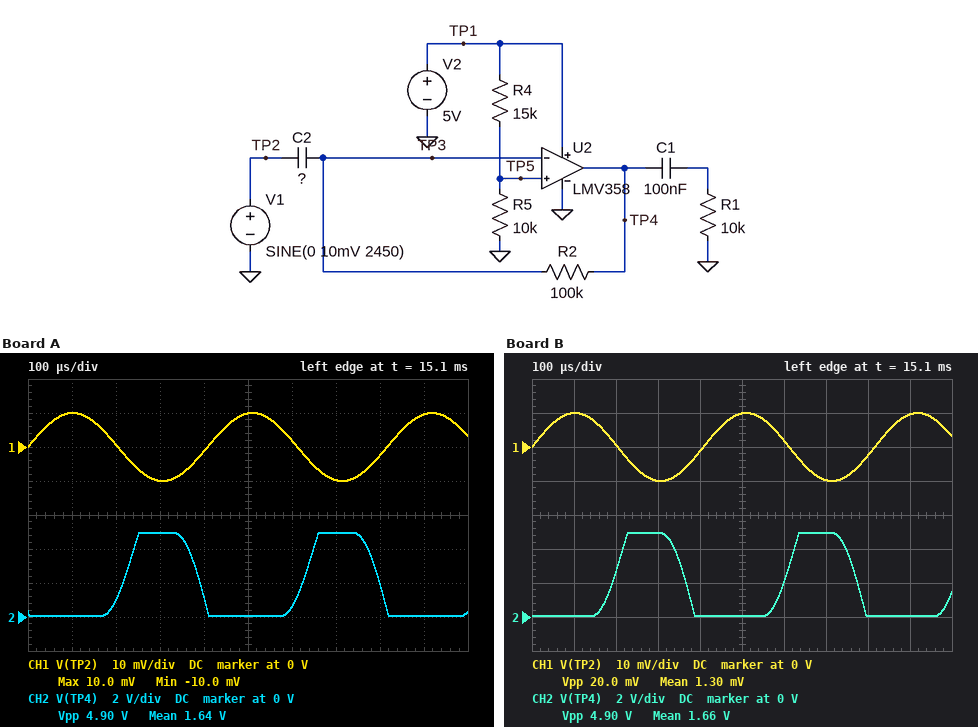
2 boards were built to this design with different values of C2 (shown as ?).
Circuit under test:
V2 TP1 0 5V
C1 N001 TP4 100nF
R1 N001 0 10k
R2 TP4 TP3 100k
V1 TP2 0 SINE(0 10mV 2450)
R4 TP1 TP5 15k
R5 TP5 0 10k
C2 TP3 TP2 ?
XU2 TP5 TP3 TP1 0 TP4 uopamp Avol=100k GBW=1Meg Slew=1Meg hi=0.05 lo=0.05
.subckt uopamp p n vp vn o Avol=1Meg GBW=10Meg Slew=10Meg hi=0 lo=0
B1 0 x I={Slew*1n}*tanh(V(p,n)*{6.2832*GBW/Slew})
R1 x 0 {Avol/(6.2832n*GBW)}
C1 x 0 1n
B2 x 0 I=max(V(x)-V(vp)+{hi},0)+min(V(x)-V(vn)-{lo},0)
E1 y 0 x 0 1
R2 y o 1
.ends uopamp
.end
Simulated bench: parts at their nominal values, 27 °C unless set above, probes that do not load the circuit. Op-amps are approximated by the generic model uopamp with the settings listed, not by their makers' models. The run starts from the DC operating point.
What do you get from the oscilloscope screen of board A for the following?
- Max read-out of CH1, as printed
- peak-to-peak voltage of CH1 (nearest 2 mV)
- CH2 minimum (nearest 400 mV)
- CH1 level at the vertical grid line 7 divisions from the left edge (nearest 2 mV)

10.0 mV
20 mV
0 V
-10 mV
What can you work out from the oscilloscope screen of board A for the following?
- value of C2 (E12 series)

150 nF
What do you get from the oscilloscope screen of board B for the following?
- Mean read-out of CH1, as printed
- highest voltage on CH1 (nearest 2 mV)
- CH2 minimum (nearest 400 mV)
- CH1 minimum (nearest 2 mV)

1.30 mV
10 mV
0 V
-10 mV
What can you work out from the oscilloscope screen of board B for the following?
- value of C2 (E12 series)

120 nF
